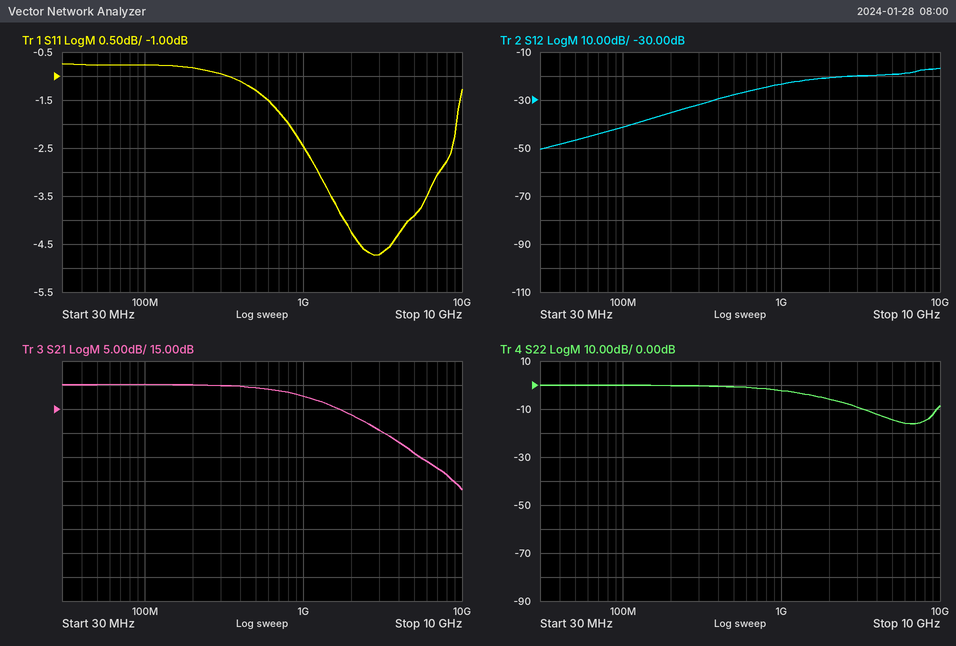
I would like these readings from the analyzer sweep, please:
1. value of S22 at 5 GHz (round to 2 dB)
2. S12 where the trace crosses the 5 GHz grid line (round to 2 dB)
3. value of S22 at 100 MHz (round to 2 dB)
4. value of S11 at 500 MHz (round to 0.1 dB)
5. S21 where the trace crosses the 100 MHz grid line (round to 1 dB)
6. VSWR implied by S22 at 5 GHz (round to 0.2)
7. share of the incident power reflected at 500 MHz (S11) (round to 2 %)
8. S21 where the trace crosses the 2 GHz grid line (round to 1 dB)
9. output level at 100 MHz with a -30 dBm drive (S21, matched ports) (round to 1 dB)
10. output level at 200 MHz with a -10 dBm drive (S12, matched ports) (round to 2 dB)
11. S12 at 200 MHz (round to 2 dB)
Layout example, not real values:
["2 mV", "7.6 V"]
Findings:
["-14 dB", "-20 dB", "0 dB", "-1.3 dB", "20 dB", "1.4", "74 %", "14 dB", "-10 dBm", "-46 dBm", "-36 dB"]
